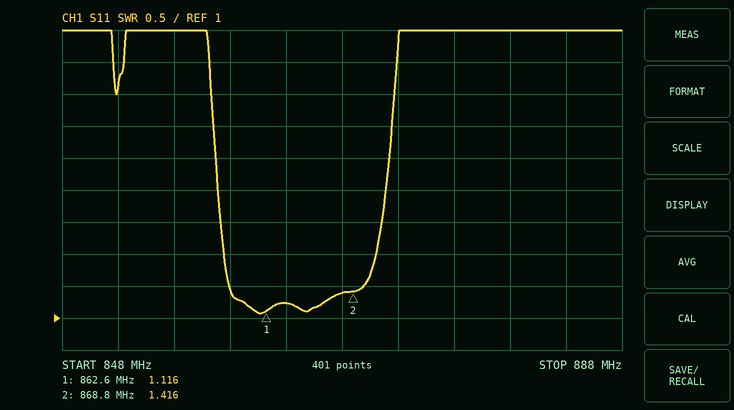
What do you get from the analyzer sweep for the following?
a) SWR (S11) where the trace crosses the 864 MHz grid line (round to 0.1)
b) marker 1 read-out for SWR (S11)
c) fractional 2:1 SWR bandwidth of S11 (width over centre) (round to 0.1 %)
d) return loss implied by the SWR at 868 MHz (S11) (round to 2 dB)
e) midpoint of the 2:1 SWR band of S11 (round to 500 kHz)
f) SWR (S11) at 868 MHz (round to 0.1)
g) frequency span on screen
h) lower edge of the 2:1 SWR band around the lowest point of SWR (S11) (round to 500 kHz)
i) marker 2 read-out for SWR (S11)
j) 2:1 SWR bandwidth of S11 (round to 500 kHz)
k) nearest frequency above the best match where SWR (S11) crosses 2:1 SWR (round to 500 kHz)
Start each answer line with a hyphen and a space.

- 1.2
- 1.116
- 1.3 %
- 16 dB
- 865.0 MHz
- 1.4
- 40 MHz
- 859.5 MHz
- 1.416
- 11.0 MHz
- 870.5 MHz
